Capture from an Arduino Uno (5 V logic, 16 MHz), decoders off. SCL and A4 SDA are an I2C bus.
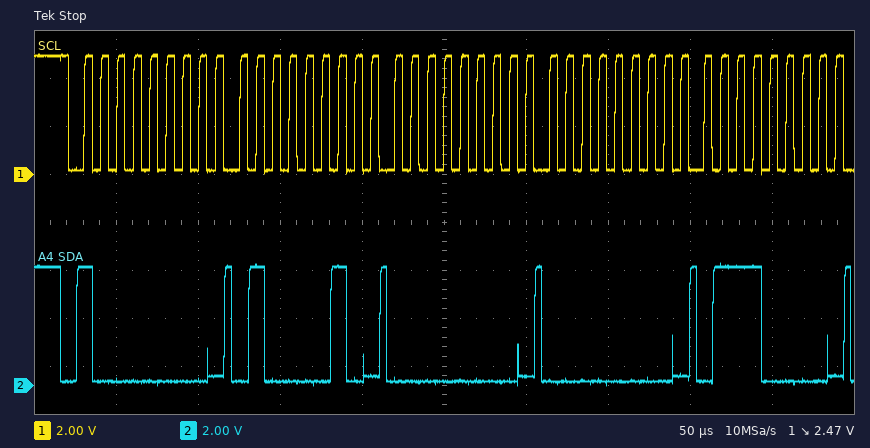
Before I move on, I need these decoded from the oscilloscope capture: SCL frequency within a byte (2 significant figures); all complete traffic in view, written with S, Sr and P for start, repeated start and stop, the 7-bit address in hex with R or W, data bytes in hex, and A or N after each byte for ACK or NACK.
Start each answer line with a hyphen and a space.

- 100 kHz
- S 40W A 42 A 00 A 00 A 70 A
